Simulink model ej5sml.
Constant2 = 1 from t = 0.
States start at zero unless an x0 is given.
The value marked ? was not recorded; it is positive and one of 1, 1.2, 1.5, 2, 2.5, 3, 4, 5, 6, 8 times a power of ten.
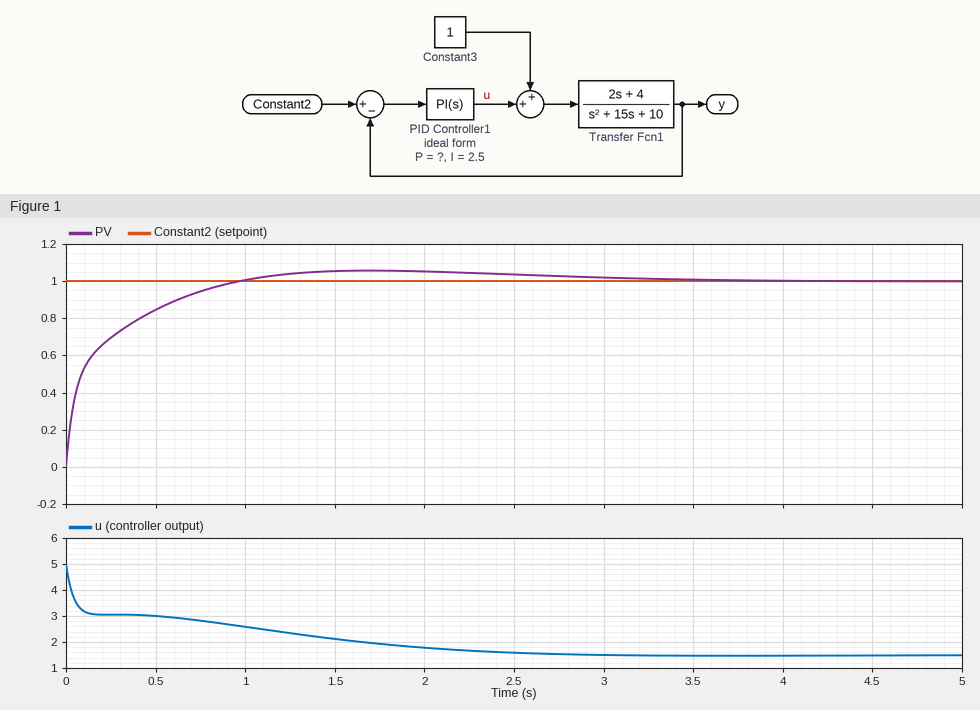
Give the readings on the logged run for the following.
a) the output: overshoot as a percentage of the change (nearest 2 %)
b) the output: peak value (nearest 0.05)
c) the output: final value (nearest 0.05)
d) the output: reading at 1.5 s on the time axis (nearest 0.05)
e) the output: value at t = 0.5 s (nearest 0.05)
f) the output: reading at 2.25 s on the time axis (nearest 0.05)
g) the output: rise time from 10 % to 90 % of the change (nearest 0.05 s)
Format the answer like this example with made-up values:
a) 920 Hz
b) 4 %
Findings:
a) 6 %
b) 1.05
c) 1.00
d) 1.05
e) 0.85
f) 1.05
g) 0.60 s
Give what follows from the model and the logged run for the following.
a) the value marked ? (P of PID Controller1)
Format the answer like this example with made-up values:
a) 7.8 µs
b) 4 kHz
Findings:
a) 5
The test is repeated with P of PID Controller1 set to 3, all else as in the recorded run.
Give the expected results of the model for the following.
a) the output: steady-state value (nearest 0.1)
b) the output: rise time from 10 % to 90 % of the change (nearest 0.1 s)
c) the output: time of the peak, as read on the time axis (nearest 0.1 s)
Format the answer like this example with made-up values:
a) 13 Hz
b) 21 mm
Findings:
a) 1.0
b) 0.9 s
c) 2.1 s
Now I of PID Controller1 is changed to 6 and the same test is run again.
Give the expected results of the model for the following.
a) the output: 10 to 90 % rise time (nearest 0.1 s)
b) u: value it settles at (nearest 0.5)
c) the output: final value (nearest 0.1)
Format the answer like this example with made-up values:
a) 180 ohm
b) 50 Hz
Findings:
a) 0.3 s
b) 1.5
c) 1.0
